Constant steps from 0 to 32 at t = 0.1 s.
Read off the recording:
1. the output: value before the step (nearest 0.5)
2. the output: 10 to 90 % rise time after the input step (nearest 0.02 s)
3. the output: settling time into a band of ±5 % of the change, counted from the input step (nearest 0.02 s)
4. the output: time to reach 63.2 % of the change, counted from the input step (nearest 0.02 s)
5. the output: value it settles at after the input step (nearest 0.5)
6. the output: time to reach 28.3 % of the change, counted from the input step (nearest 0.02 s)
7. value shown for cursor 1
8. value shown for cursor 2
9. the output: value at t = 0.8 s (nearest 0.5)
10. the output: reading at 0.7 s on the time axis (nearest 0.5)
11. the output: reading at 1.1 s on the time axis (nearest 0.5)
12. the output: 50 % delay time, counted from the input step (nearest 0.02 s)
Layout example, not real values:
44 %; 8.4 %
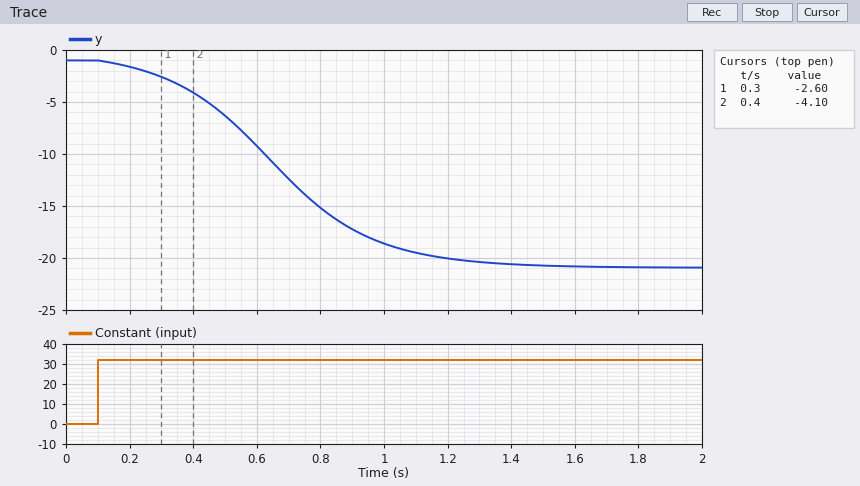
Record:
-1.0; 0.70 s; 1.08 s; 0.64 s; -21.0; 0.42 s; -2.60; -4.10; -15.0; -12.5; -19.5; 0.56 s
